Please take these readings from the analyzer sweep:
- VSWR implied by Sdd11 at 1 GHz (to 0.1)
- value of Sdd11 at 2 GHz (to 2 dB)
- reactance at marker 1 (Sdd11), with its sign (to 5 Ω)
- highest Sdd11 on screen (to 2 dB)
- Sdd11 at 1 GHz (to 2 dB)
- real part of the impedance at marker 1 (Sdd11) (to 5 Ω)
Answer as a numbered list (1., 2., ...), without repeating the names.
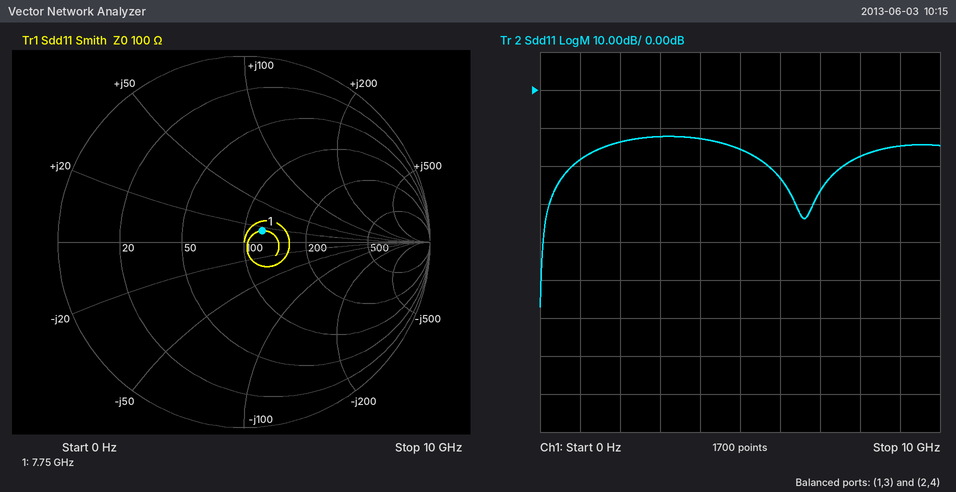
1. 1.3
2. -14 dB
3. +15 Ω
4. -12 dB
5. -18 dB
6. 120 Ω
